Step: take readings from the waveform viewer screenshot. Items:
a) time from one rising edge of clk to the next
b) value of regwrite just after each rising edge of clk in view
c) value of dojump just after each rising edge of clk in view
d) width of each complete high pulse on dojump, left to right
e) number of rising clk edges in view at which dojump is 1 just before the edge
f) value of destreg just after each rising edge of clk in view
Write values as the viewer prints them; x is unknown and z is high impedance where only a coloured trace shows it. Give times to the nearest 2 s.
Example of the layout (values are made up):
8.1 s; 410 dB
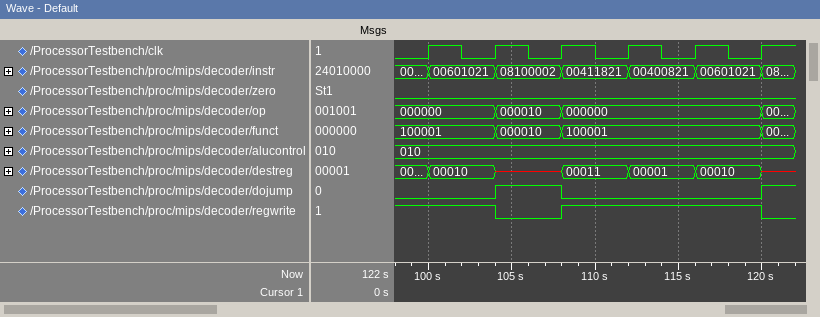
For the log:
4 s; 1 0 1 1 1 0; 0 1 0 0 0 1; 4 s; 1; 00010, x, 00011, 00001, 00010, x
